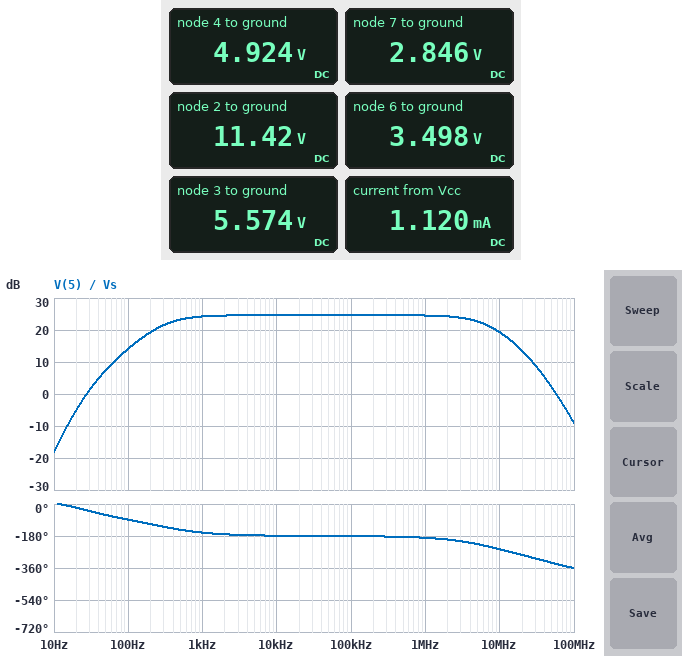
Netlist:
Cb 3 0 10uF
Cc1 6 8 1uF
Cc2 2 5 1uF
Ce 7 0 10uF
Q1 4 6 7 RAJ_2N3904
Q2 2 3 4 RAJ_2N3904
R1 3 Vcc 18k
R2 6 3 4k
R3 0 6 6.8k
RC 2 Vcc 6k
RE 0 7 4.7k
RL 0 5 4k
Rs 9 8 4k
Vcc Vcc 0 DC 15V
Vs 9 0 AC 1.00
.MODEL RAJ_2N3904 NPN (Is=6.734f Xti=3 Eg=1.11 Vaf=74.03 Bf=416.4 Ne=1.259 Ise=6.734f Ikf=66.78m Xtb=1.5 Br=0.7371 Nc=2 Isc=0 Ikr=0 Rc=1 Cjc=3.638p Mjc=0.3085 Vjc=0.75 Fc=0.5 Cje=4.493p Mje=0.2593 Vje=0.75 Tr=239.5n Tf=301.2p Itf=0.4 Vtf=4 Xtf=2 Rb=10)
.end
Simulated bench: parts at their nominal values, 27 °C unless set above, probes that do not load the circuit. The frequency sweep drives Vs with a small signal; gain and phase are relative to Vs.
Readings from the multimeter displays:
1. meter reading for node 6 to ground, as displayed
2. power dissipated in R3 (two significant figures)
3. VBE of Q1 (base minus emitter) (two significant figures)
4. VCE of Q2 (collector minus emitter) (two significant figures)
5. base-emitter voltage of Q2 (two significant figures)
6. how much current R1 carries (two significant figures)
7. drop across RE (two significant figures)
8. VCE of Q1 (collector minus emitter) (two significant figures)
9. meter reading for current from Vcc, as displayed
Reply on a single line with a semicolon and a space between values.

3.498 V; 1.8 mW; 650 mV; 6.5 V; 650 mV; 520 µA; 2.8 V; 2.1 V; 1.120 mA
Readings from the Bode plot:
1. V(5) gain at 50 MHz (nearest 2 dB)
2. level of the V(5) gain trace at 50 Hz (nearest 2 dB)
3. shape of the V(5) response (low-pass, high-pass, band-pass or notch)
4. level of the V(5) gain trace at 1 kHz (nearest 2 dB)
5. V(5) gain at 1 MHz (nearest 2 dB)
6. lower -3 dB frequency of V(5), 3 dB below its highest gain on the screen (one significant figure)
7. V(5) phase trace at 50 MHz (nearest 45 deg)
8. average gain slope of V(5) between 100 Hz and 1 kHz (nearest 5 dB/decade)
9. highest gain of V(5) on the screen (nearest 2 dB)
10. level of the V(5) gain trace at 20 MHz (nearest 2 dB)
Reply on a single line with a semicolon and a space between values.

2 dB; 8 dB; band-pass; 24 dB; 24 dB; 300 Hz; -315 deg; 10 dB/decade; 24 dB; 14 dB
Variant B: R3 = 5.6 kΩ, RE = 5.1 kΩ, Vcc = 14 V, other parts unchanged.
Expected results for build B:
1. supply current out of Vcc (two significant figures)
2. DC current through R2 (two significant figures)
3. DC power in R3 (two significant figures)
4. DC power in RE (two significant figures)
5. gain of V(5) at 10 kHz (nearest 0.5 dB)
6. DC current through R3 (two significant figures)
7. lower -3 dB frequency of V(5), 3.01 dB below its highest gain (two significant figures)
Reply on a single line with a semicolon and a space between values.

930 µA; 510 µA; 1.4 mW; 920 µW; 21.5 dB; 500 µA; 230 Hz
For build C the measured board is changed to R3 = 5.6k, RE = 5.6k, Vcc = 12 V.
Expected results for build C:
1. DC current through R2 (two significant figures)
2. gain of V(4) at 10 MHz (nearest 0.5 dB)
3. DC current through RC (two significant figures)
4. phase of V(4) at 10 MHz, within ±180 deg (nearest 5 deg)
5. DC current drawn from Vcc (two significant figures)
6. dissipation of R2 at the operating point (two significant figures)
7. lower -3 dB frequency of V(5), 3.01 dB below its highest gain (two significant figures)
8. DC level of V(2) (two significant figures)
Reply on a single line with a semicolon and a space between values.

430 µA; -14.0 dB; 310 µA; 125 deg; 750 µA; 750 µW; 180 Hz; 10 V
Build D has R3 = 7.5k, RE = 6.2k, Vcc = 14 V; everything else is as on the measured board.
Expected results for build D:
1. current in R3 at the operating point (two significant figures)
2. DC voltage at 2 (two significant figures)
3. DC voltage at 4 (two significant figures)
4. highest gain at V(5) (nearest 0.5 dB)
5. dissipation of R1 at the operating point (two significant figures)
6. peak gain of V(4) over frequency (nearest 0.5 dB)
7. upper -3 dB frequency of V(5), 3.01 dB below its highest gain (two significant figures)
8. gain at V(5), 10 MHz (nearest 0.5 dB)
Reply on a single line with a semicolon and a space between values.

470 µA; 11 V; 4.8 V; 23.0 dB; 4.1 mW; -9.5 dB; 6.7 MHz; 17.5 dB
